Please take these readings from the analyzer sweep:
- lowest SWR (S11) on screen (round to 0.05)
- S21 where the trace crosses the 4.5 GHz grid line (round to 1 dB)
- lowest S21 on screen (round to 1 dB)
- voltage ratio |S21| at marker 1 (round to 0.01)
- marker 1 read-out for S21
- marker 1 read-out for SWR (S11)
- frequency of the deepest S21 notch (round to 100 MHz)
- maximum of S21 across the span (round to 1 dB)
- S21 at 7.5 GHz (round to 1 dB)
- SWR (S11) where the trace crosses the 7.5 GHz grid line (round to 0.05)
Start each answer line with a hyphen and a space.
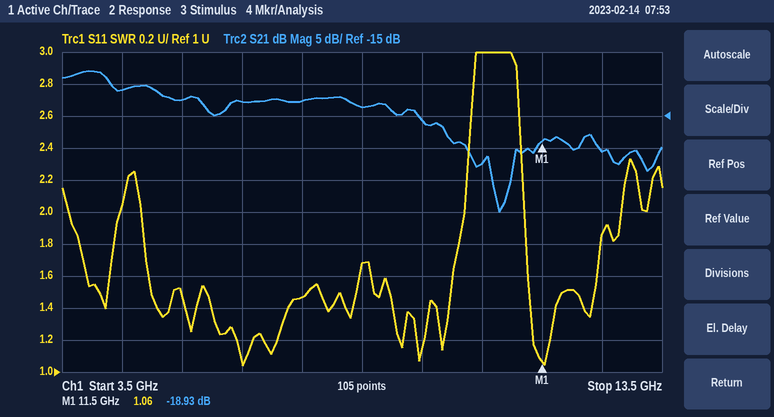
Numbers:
- 1.05
- -11 dB
- -30 dB
- 0.11
- -18.93 dB
- 1.06
- 10.8 GHz
- -8 dB
- -13 dB
- 1.45
